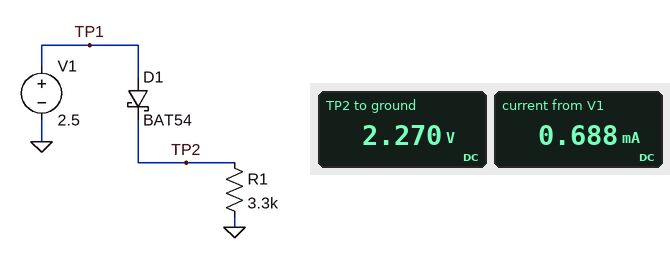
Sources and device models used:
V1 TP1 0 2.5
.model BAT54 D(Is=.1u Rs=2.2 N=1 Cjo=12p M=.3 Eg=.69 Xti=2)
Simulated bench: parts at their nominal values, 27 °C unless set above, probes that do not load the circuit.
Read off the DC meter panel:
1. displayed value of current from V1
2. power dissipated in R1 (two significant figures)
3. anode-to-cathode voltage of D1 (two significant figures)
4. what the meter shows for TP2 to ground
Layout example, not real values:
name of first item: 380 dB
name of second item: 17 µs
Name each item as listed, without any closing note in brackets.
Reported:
displayed value of current from V1: 0.688 mA
power dissipated in R1: 1.6 mW
anode-to-cathode voltage of D1: 230 mV
what the meter shows for TP2 to ground: 2.270 V
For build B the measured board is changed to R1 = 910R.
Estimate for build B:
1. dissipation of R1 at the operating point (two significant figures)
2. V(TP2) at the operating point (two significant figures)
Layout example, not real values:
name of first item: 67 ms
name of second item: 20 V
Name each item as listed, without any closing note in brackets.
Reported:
dissipation of R1 at the operating point: 5.5 mW
V(TP2) at the operating point: 2.2 V
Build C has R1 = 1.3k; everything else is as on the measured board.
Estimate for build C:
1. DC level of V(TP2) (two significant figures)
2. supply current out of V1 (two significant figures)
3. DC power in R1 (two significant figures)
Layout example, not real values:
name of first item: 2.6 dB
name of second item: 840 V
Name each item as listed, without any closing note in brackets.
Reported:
DC level of V(TP2): 2.2 V
supply current out of V1: 1.7 mA
DC power in R1: 3.9 mW
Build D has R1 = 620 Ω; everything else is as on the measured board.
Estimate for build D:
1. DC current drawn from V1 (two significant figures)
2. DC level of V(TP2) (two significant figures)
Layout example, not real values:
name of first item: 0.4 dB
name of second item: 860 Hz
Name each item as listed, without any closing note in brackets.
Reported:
DC current drawn from V1: 3.6 mA
DC level of V(TP2): 2.2 V
